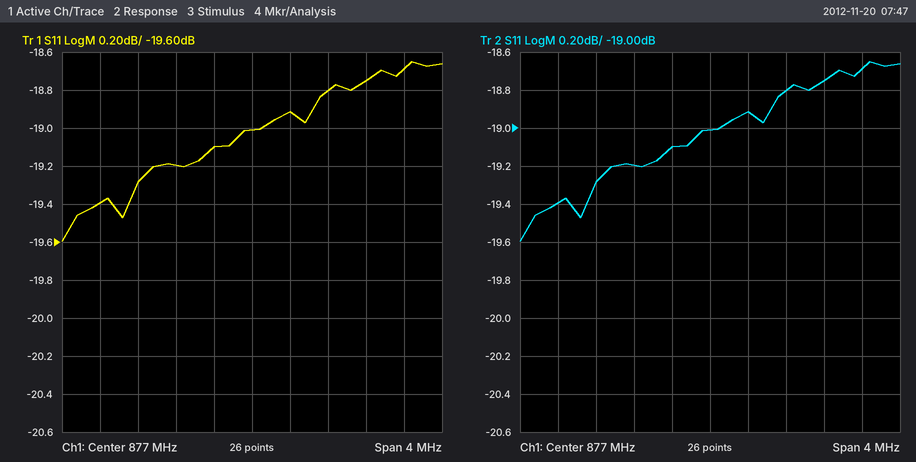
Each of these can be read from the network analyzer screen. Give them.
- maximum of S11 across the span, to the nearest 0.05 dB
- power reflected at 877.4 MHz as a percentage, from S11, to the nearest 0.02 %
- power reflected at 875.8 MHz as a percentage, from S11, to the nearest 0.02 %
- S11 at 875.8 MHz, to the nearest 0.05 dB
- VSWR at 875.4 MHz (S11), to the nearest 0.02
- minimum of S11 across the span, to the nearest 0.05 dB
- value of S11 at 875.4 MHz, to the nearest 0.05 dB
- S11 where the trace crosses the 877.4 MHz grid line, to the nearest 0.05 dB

-18.65 dB
1.28 %
1.18 %
-19.30 dB
1.24
-19.60 dB
-19.40 dB
-18.90 dB
